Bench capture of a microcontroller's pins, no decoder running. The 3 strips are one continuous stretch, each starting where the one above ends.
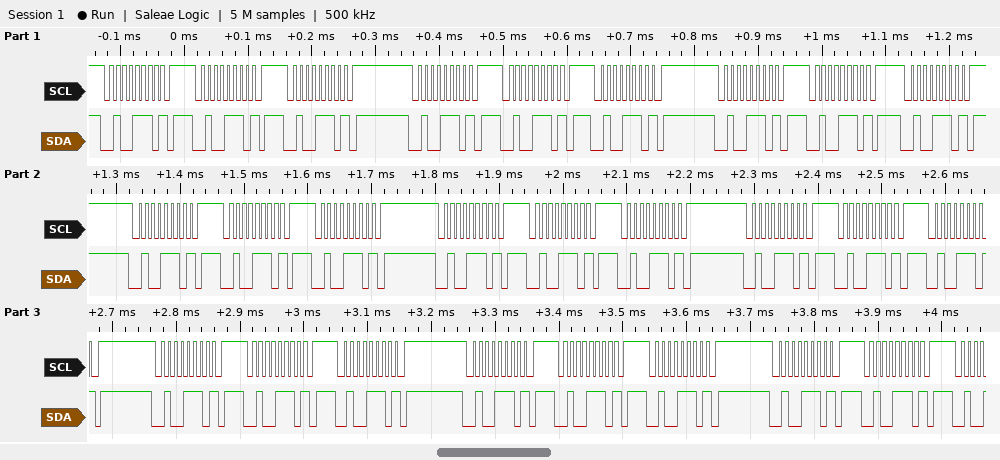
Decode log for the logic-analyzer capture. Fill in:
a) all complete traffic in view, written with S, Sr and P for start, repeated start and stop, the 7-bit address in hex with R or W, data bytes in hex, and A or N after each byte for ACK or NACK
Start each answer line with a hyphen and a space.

- S 27W N P S 27W N P S 27W N P S 27W N P S 27W N P S 27W N P S 27W N P S 27W N P S 27W N P S 27W N P S 27W N P S 27W N P S 27W N P S 27W N P S 27W N P S 27W N P S 27W N P S 27W N P S 27W N P S 27W N P S 27W N P S 27W N P S 27W N P S 27W N P S 27W N P S 27W N P
